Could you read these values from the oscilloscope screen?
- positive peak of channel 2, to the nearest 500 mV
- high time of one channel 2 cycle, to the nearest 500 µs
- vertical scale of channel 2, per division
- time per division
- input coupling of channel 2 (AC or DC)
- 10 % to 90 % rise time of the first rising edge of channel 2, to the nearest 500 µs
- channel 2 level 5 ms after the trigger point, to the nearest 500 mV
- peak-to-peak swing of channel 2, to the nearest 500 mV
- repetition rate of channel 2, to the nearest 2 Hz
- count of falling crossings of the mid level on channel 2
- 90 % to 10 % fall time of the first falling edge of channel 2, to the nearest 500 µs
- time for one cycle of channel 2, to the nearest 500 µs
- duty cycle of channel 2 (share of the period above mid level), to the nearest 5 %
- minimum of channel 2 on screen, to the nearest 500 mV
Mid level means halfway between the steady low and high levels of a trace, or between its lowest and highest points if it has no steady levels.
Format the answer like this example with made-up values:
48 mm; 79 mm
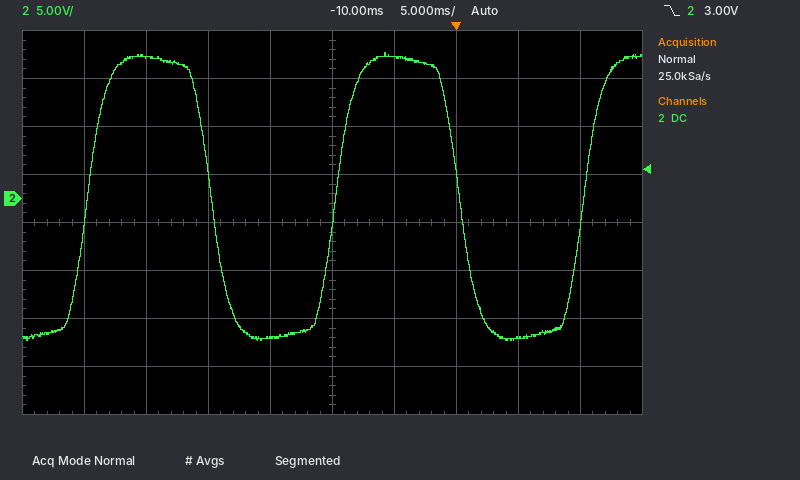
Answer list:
15.0 V; 10.0 ms; 5 V; 5 ms; DC; 3.0 ms; -14.5 V; 30.0 V; 50 Hz; 2; 3.0 ms; 20.0 ms; 50 %; -15.0 V
